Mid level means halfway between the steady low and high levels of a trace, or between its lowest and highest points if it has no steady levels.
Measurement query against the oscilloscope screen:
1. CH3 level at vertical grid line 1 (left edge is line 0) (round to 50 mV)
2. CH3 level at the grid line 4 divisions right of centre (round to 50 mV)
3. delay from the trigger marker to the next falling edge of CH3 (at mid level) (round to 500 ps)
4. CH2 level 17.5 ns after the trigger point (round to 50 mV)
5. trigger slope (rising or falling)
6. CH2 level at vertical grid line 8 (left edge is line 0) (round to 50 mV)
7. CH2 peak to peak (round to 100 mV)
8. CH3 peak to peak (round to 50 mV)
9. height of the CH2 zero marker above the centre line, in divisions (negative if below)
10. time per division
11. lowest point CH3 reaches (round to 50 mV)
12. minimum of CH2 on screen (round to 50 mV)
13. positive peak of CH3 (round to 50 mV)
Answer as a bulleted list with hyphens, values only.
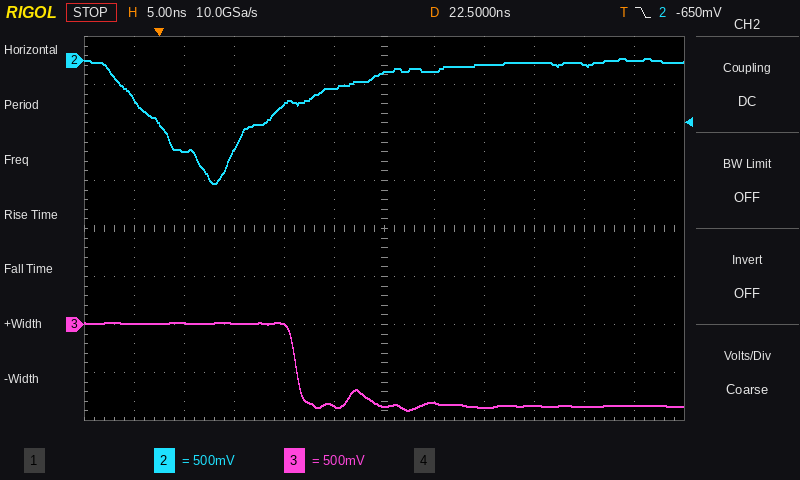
- 0 mV
- -850 mV
- 13.5 ns
- -300 mV
- falling
- -50 mV
- 1.30 V
- 900 mV
- +3.5 div
- 5 ns
- -900 mV
- -1.30 V
- 0 mV
